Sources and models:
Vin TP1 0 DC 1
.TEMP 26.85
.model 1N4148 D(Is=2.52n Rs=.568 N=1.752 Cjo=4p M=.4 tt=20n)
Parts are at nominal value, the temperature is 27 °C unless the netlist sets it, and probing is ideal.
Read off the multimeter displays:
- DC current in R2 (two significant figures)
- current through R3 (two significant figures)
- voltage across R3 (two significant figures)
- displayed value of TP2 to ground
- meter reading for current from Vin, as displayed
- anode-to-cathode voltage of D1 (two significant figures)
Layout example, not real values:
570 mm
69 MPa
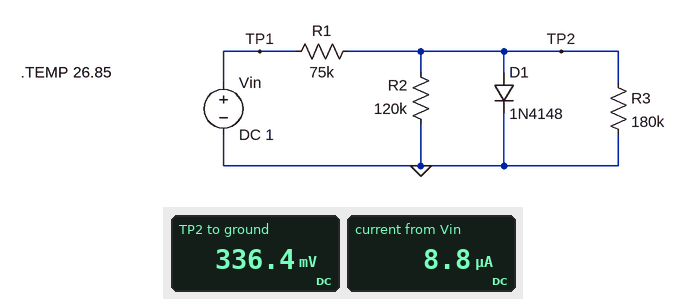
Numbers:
2.8 µA
1.9 µA
340 mV
336.4 mV
8.8 µA
340 mV
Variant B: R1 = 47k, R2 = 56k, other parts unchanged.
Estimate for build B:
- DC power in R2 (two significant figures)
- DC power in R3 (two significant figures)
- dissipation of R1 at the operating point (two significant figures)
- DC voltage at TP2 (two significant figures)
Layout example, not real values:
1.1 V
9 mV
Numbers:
2.2 µW
680 nW
9.0 µW
350 mV
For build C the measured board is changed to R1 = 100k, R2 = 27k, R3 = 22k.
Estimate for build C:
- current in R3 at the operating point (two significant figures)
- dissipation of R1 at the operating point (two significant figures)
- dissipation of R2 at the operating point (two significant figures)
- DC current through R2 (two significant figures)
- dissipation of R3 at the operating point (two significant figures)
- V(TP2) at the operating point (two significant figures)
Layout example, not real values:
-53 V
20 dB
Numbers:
4.9 µA
8.0 µW
430 nW
4.0 µA
530 nW
110 mV
